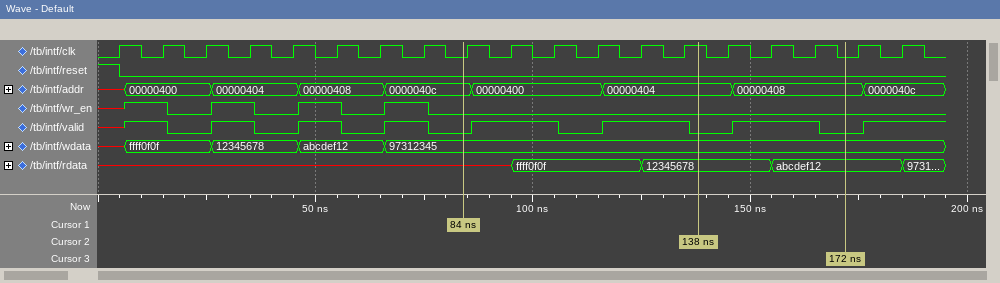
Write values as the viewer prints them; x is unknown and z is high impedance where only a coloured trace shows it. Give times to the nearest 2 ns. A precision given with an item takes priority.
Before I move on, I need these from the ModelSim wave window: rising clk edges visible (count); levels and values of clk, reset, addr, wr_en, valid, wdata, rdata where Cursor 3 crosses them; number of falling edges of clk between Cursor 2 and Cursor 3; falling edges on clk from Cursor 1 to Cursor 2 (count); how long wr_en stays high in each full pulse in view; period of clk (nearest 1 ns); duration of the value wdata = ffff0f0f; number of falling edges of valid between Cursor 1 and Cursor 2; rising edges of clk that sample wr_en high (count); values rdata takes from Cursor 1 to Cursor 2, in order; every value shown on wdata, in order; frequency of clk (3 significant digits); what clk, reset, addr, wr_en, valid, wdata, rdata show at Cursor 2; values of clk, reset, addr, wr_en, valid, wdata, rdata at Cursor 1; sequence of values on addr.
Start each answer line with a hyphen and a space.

- 19
- clk=0, reset=0, addr=00000408, wr_en=0, valid=0, wdata=97312345, rdata=abcdef12
- 4
- 5
- 10 ns, 10 ns, 10 ns
- 10 ns
- 20 ns
- 2
- 4
- x, ffff0f0f, 12345678
- x, ffff0f0f, 12345678, abcdef12, 97312345
- 100 MHz
- clk=1, reset=0, addr=00000404, wr_en=0, valid=0, wdata=97312345, rdata=12345678
- clk=0, reset=0, addr=0000040c, wr_en=0, valid=0, wdata=97312345, rdata=x
- x, 00000400, 00000404, 00000408, 0000040c, 00000400, 00000404, 00000408, 0000040c
